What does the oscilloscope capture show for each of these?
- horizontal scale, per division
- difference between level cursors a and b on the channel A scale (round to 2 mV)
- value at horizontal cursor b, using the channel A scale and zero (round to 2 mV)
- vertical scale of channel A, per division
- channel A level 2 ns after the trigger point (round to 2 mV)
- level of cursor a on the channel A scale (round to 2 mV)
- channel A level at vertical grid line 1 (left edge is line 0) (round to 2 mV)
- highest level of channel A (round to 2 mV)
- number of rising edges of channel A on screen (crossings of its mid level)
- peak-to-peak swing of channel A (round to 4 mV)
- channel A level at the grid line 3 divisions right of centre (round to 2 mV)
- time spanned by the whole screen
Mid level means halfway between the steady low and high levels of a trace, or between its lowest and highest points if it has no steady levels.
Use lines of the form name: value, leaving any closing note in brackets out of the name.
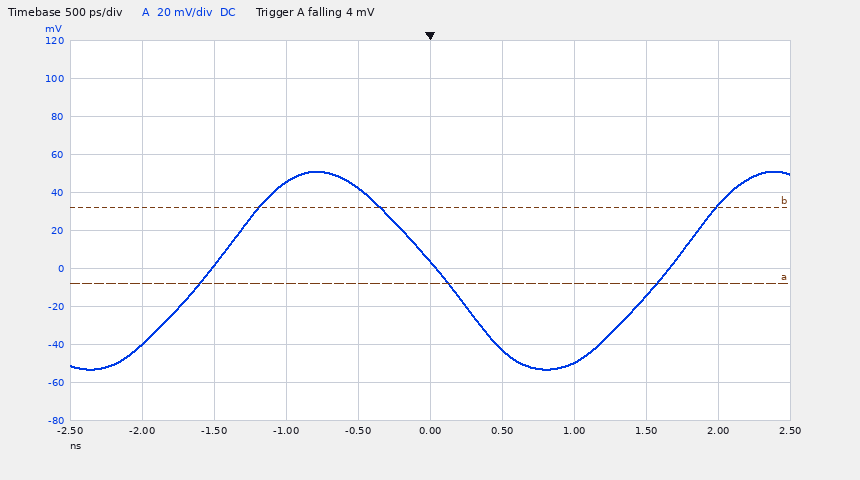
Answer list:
horizontal scale, per division: 500 ps
difference between level cursors a and b on the channel A scale: 40 mV
value at horizontal cursor b, using the channel A scale and zero: 32 mV
vertical scale of channel A, per division: 20 mV
channel A level 2 ns after the trigger point: 34 mV
level of cursor a on the channel A scale: -8 mV
channel A level at vertical grid line 1 (left edge is line 0): -40 mV
highest level of channel A: 52 mV
number of rising edges of channel A on screen: 2
peak-to-peak swing of channel A: 104 mV
channel A level at the grid line 3 divisions right of centre: -14 mV
time spanned by the whole screen: 5 ns
